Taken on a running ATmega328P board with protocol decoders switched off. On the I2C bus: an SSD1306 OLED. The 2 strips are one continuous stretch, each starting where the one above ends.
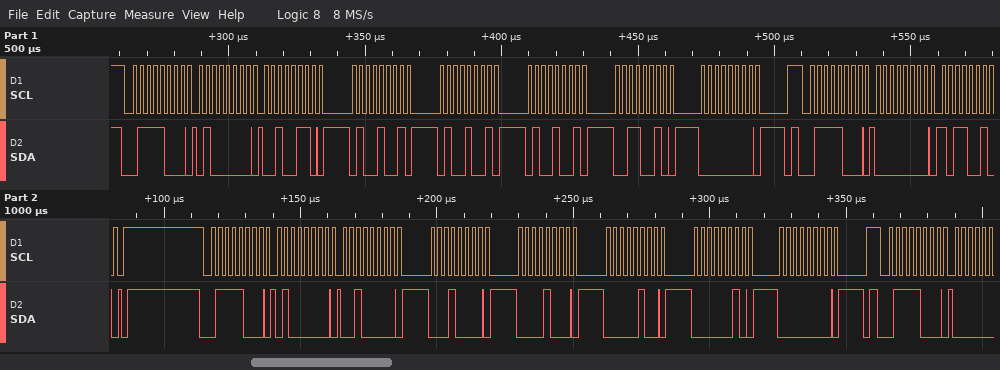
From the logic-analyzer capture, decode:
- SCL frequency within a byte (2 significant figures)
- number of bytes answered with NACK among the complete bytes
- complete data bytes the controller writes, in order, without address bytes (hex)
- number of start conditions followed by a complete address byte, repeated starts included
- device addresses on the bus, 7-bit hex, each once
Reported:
400 kHz
0
40 26 49 49 49 32 00 00 B2 40 20 10 08 04 02 00
4
0x3C
